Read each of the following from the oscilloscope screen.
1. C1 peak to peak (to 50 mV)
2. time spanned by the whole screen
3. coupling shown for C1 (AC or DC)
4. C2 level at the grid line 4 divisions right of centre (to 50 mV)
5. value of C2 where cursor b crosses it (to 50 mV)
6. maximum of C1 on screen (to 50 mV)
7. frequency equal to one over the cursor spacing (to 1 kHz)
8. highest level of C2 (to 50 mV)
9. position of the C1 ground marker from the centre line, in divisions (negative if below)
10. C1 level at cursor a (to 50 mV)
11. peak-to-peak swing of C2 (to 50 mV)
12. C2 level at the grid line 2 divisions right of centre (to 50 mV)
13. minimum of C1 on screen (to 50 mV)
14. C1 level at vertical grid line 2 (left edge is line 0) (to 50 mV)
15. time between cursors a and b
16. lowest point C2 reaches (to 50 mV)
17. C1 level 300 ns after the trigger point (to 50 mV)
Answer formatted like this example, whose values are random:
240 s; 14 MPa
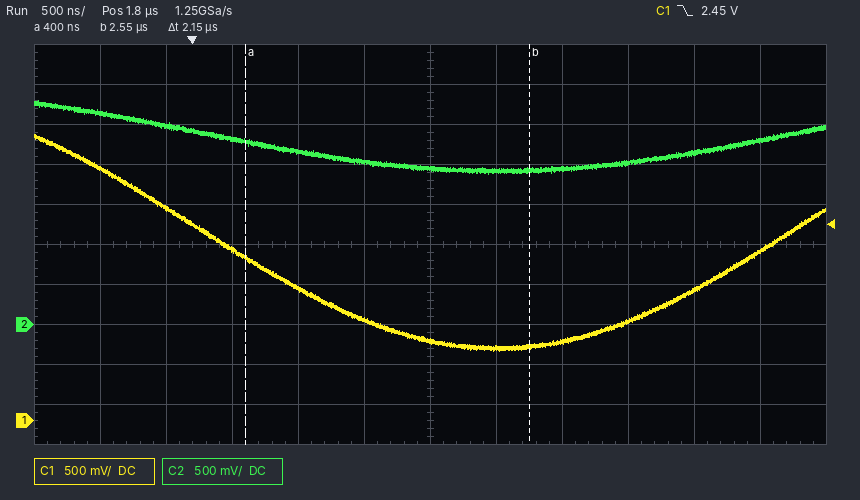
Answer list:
2.70 V; 6 µs; DC; 2.15 V; 1.95 V; 3.60 V; 465 kHz; 2.80 V; -4.4 div; 2.05 V; 900 mV; 1.95 V; 900 mV; 2.65 V; 2.15 µs; 1.90 V; 2.15 V
